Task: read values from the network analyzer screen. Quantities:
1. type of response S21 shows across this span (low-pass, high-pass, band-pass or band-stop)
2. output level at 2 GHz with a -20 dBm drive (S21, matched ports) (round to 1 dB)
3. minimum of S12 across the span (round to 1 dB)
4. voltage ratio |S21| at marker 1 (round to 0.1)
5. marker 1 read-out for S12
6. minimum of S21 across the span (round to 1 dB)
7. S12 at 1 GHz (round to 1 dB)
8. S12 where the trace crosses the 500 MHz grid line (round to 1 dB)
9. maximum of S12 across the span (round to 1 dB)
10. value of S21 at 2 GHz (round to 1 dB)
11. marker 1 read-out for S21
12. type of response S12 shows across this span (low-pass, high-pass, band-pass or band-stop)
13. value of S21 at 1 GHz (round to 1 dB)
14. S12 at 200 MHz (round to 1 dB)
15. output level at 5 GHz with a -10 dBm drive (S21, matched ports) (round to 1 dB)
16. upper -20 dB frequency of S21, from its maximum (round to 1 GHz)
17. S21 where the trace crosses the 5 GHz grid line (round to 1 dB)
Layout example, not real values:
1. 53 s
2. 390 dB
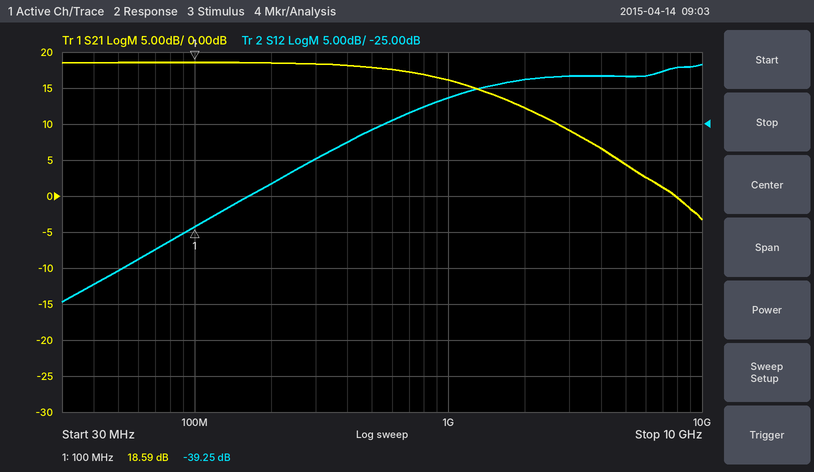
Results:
1. low-pass
2. -8 dBm
3. -50 dB
4. 8.5
5. -39.25 dB
6. -3 dB
7. -21 dB
8. -26 dB
9. -17 dB
10. 12 dB
11. 18.59 dB
12. high-pass
13. 16 dB
14. -33 dB
15. -6 dBm
16. 9 GHz
17. 4 dB
